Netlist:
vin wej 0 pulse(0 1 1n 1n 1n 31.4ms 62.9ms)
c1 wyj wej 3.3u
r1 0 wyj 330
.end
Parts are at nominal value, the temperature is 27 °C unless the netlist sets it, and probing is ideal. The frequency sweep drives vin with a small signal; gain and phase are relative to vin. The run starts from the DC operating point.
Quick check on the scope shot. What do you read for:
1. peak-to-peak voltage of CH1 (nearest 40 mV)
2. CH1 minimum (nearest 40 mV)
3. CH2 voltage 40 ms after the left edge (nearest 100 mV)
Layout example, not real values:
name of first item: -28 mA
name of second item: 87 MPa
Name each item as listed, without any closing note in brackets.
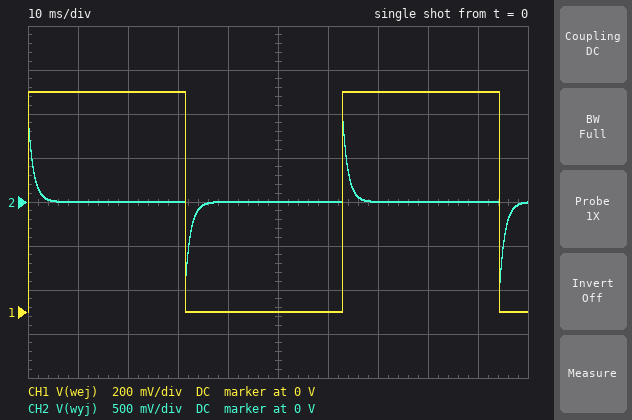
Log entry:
peak-to-peak voltage of CH1: 1.00 V
CH1 minimum: 0 V
CH2 voltage 40 ms after the left edge: 0 V
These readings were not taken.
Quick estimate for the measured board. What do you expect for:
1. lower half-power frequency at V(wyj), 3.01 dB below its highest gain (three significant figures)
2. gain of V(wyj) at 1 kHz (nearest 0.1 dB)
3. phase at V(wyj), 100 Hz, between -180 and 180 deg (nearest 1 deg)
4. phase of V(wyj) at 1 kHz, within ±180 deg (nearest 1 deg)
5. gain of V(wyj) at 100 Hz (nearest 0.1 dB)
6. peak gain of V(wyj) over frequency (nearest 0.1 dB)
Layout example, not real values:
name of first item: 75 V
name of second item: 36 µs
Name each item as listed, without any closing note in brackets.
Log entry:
lower half-power frequency at V(wyj), 3.01 dB below its highest gain: 146 Hz
gain of V(wyj) at 1 kHz: -0.1 dB
phase at V(wyj), 100 Hz, between -180 and 180 deg: 56 deg
phase of V(wyj) at 1 kHz, within ±180 deg: 8 deg
gain of V(wyj) at 100 Hz: -5.0 dB
peak gain of V(wyj) over frequency: 0 dB
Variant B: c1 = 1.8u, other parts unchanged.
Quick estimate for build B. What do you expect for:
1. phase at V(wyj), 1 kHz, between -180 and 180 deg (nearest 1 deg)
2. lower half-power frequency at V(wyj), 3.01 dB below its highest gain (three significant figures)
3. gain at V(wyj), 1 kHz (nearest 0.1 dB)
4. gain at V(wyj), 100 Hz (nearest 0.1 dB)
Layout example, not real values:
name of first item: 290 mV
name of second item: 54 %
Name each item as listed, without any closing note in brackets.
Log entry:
phase at V(wyj), 1 kHz, between -180 and 180 deg: 15 deg
lower half-power frequency at V(wyj), 3.01 dB below its highest gain: 268 Hz
gain at V(wyj), 1 kHz: -0.3 dB
gain at V(wyj), 100 Hz: -9.1 dB
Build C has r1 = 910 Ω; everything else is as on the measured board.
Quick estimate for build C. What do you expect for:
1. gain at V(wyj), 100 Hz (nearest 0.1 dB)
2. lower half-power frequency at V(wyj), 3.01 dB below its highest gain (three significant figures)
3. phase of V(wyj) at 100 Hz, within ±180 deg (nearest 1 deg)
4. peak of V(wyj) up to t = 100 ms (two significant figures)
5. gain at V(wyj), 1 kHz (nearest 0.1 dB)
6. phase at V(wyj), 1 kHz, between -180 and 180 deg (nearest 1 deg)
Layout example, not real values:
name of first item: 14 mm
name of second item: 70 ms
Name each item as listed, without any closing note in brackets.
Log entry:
gain at V(wyj), 100 Hz: -1.1 dB
lower half-power frequency at V(wyj), 3.01 dB below its highest gain: 53.0 Hz
phase of V(wyj) at 100 Hz, within ±180 deg: 28 deg
peak of V(wyj) up to t = 100 ms: 1.0 V
gain at V(wyj), 1 kHz: 0 dB
phase at V(wyj), 1 kHz, between -180 and 180 deg: 3 deg
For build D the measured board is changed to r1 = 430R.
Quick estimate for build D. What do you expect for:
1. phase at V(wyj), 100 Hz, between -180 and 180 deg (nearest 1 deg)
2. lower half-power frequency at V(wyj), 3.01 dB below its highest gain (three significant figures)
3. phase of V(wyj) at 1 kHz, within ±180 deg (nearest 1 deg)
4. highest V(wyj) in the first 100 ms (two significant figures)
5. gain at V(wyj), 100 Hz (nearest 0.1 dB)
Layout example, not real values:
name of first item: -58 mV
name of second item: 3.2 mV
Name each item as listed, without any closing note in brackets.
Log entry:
phase at V(wyj), 100 Hz, between -180 and 180 deg: 48 deg
lower half-power frequency at V(wyj), 3.01 dB below its highest gain: 112 Hz
phase of V(wyj) at 1 kHz, within ±180 deg: 6 deg
highest V(wyj) in the first 100 ms: 1.0 V
gain at V(wyj), 100 Hz: -3.5 dB
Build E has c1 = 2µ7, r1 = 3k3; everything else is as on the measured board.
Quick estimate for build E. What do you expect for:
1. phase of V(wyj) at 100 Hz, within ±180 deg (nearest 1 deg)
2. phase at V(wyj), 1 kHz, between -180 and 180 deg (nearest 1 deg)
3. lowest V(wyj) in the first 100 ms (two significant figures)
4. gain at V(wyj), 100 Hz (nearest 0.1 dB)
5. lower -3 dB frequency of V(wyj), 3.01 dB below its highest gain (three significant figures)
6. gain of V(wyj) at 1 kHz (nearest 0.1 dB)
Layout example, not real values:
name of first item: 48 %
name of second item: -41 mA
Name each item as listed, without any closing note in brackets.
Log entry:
phase of V(wyj) at 100 Hz, within ±180 deg: 10 deg
phase at V(wyj), 1 kHz, between -180 and 180 deg: 1 deg
lowest V(wyj) in the first 100 ms: -970 mV
gain at V(wyj), 100 Hz: -0.1 dB
lower -3 dB frequency of V(wyj), 3.01 dB below its highest gain: 17.9 Hz
gain of V(wyj) at 1 kHz: 0 dB
